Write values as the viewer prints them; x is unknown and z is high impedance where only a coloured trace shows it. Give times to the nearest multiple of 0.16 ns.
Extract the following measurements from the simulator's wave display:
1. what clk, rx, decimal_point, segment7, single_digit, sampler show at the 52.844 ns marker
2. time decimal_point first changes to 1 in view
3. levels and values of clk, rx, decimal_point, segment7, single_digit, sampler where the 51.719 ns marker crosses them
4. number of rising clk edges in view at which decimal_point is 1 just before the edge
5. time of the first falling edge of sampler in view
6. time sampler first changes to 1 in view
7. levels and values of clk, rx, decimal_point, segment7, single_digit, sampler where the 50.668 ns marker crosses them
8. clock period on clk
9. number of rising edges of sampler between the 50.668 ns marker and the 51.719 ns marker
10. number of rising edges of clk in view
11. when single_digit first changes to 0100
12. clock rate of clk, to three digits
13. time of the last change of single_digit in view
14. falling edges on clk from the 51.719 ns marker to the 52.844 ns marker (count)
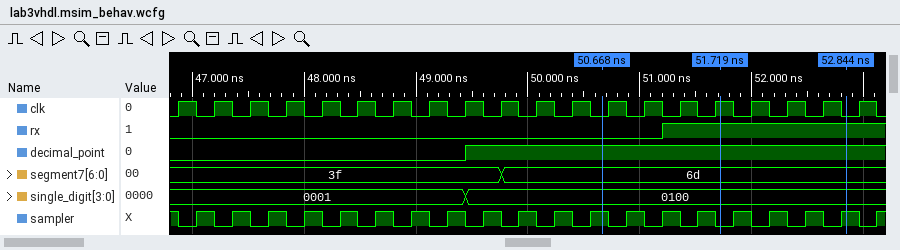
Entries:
clk=0, rx=1, decimal_point=1, segment7=6d, single_digit=0100, sampler=1
49.44 ns
clk=1, rx=1, decimal_point=1, segment7=6d, single_digit=0100, sampler=0
11
46.88 ns
47.04 ns
clk=0, rx=0, decimal_point=1, segment7=6d, single_digit=0100, sampler=1
0.32 ns
3
20
49.44 ns
3.12 GHz
49.44 ns
4
